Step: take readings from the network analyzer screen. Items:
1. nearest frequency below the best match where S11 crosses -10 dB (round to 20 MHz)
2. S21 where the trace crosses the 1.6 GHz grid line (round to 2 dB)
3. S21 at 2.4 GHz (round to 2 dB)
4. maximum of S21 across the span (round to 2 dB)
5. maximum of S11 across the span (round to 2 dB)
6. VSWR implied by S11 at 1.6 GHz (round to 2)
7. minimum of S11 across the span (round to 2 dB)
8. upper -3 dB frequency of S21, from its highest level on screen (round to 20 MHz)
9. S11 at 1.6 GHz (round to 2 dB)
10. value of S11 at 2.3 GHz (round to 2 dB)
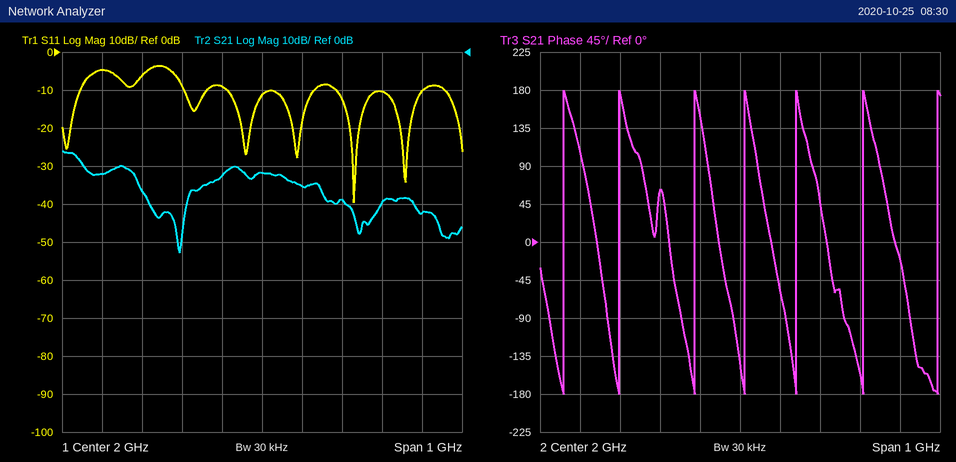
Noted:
2.18 GHz
-32 dB
-42 dB
-26 dB
-4 dB
4
-40 dB
1.54 GHz
-4 dB
-10 dB
